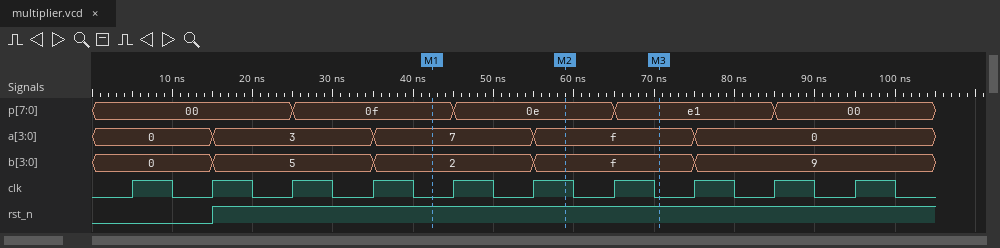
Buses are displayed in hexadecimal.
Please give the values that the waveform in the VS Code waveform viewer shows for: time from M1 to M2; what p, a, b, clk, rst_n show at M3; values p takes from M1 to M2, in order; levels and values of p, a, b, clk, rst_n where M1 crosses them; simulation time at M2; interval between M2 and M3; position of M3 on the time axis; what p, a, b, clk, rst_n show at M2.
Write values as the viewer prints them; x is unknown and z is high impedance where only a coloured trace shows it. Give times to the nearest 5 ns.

15 ns
p=e1, a=f, b=f, clk=0, rst_n=1
0f, 0e
p=0f, a=7, b=2, clk=0, rst_n=1
60 ns
10 ns
70 ns
p=0e, a=f, b=f, clk=1, rst_n=1
